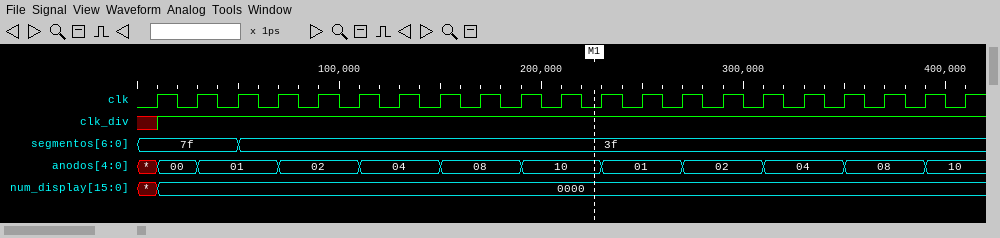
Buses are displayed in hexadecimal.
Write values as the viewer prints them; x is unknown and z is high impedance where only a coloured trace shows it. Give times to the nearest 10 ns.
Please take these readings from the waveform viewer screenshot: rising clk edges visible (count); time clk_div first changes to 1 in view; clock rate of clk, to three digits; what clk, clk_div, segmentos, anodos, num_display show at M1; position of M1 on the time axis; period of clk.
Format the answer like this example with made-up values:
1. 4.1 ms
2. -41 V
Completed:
1. 21
2. 10 ns
3. 50.0 MHz
4. clk=0, clk_div=1, segmentos=3f, anodos=10, num_display=0000
5. 230 ns
6. 20 ns
